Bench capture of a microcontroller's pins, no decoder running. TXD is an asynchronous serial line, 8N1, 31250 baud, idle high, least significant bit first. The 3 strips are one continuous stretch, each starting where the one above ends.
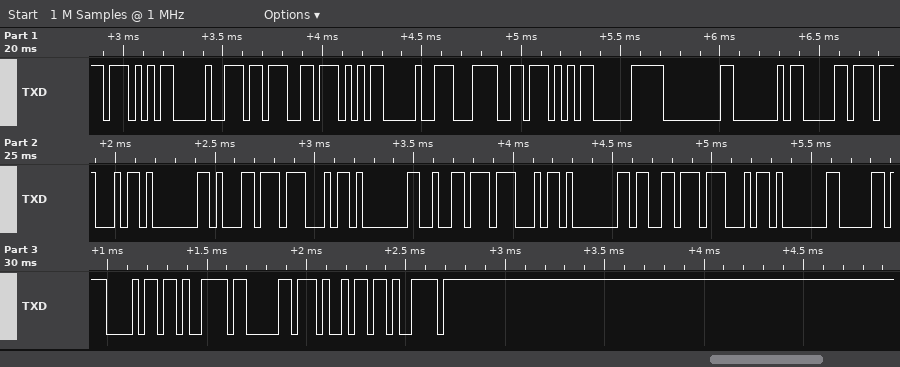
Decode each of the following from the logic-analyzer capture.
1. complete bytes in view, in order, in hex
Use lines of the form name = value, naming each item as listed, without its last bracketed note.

complete bytes in view, in order, in hex = 0x57 0x90 0x3B 0x57 0x90 0x3C 0x57 0xE0 0x00 0x40 0xB0 0x47 0x01 0xB1 0x47 0x01 0xB2 0x47 0x01 0xB3 0x47 0x01 0xB0 0x68 0x79 0xB0 0x69 0x79
